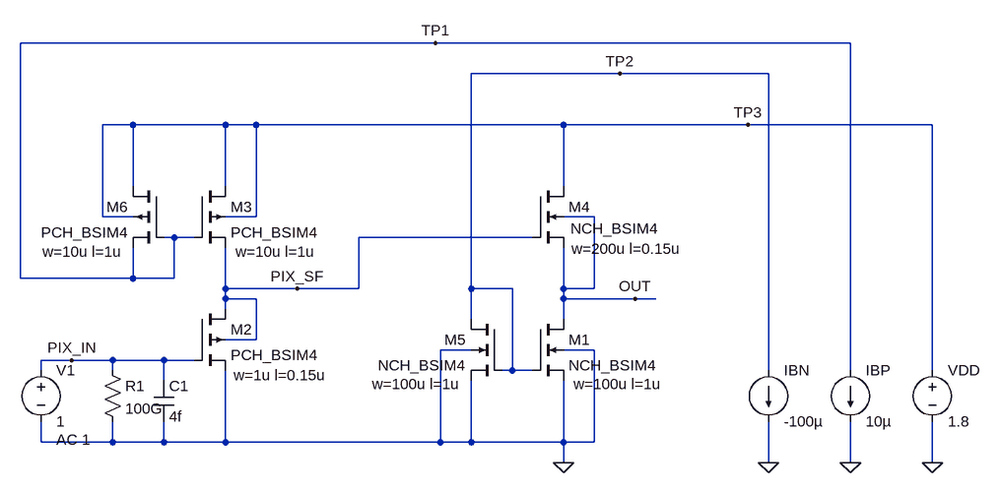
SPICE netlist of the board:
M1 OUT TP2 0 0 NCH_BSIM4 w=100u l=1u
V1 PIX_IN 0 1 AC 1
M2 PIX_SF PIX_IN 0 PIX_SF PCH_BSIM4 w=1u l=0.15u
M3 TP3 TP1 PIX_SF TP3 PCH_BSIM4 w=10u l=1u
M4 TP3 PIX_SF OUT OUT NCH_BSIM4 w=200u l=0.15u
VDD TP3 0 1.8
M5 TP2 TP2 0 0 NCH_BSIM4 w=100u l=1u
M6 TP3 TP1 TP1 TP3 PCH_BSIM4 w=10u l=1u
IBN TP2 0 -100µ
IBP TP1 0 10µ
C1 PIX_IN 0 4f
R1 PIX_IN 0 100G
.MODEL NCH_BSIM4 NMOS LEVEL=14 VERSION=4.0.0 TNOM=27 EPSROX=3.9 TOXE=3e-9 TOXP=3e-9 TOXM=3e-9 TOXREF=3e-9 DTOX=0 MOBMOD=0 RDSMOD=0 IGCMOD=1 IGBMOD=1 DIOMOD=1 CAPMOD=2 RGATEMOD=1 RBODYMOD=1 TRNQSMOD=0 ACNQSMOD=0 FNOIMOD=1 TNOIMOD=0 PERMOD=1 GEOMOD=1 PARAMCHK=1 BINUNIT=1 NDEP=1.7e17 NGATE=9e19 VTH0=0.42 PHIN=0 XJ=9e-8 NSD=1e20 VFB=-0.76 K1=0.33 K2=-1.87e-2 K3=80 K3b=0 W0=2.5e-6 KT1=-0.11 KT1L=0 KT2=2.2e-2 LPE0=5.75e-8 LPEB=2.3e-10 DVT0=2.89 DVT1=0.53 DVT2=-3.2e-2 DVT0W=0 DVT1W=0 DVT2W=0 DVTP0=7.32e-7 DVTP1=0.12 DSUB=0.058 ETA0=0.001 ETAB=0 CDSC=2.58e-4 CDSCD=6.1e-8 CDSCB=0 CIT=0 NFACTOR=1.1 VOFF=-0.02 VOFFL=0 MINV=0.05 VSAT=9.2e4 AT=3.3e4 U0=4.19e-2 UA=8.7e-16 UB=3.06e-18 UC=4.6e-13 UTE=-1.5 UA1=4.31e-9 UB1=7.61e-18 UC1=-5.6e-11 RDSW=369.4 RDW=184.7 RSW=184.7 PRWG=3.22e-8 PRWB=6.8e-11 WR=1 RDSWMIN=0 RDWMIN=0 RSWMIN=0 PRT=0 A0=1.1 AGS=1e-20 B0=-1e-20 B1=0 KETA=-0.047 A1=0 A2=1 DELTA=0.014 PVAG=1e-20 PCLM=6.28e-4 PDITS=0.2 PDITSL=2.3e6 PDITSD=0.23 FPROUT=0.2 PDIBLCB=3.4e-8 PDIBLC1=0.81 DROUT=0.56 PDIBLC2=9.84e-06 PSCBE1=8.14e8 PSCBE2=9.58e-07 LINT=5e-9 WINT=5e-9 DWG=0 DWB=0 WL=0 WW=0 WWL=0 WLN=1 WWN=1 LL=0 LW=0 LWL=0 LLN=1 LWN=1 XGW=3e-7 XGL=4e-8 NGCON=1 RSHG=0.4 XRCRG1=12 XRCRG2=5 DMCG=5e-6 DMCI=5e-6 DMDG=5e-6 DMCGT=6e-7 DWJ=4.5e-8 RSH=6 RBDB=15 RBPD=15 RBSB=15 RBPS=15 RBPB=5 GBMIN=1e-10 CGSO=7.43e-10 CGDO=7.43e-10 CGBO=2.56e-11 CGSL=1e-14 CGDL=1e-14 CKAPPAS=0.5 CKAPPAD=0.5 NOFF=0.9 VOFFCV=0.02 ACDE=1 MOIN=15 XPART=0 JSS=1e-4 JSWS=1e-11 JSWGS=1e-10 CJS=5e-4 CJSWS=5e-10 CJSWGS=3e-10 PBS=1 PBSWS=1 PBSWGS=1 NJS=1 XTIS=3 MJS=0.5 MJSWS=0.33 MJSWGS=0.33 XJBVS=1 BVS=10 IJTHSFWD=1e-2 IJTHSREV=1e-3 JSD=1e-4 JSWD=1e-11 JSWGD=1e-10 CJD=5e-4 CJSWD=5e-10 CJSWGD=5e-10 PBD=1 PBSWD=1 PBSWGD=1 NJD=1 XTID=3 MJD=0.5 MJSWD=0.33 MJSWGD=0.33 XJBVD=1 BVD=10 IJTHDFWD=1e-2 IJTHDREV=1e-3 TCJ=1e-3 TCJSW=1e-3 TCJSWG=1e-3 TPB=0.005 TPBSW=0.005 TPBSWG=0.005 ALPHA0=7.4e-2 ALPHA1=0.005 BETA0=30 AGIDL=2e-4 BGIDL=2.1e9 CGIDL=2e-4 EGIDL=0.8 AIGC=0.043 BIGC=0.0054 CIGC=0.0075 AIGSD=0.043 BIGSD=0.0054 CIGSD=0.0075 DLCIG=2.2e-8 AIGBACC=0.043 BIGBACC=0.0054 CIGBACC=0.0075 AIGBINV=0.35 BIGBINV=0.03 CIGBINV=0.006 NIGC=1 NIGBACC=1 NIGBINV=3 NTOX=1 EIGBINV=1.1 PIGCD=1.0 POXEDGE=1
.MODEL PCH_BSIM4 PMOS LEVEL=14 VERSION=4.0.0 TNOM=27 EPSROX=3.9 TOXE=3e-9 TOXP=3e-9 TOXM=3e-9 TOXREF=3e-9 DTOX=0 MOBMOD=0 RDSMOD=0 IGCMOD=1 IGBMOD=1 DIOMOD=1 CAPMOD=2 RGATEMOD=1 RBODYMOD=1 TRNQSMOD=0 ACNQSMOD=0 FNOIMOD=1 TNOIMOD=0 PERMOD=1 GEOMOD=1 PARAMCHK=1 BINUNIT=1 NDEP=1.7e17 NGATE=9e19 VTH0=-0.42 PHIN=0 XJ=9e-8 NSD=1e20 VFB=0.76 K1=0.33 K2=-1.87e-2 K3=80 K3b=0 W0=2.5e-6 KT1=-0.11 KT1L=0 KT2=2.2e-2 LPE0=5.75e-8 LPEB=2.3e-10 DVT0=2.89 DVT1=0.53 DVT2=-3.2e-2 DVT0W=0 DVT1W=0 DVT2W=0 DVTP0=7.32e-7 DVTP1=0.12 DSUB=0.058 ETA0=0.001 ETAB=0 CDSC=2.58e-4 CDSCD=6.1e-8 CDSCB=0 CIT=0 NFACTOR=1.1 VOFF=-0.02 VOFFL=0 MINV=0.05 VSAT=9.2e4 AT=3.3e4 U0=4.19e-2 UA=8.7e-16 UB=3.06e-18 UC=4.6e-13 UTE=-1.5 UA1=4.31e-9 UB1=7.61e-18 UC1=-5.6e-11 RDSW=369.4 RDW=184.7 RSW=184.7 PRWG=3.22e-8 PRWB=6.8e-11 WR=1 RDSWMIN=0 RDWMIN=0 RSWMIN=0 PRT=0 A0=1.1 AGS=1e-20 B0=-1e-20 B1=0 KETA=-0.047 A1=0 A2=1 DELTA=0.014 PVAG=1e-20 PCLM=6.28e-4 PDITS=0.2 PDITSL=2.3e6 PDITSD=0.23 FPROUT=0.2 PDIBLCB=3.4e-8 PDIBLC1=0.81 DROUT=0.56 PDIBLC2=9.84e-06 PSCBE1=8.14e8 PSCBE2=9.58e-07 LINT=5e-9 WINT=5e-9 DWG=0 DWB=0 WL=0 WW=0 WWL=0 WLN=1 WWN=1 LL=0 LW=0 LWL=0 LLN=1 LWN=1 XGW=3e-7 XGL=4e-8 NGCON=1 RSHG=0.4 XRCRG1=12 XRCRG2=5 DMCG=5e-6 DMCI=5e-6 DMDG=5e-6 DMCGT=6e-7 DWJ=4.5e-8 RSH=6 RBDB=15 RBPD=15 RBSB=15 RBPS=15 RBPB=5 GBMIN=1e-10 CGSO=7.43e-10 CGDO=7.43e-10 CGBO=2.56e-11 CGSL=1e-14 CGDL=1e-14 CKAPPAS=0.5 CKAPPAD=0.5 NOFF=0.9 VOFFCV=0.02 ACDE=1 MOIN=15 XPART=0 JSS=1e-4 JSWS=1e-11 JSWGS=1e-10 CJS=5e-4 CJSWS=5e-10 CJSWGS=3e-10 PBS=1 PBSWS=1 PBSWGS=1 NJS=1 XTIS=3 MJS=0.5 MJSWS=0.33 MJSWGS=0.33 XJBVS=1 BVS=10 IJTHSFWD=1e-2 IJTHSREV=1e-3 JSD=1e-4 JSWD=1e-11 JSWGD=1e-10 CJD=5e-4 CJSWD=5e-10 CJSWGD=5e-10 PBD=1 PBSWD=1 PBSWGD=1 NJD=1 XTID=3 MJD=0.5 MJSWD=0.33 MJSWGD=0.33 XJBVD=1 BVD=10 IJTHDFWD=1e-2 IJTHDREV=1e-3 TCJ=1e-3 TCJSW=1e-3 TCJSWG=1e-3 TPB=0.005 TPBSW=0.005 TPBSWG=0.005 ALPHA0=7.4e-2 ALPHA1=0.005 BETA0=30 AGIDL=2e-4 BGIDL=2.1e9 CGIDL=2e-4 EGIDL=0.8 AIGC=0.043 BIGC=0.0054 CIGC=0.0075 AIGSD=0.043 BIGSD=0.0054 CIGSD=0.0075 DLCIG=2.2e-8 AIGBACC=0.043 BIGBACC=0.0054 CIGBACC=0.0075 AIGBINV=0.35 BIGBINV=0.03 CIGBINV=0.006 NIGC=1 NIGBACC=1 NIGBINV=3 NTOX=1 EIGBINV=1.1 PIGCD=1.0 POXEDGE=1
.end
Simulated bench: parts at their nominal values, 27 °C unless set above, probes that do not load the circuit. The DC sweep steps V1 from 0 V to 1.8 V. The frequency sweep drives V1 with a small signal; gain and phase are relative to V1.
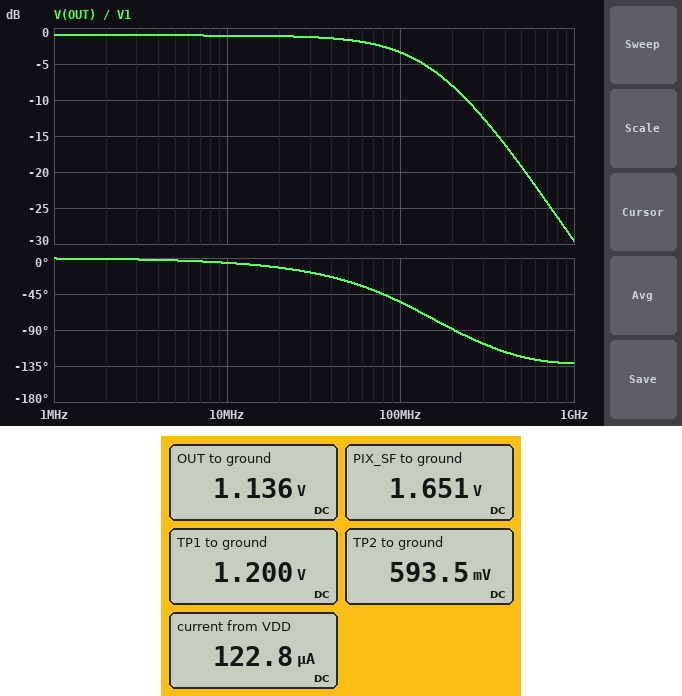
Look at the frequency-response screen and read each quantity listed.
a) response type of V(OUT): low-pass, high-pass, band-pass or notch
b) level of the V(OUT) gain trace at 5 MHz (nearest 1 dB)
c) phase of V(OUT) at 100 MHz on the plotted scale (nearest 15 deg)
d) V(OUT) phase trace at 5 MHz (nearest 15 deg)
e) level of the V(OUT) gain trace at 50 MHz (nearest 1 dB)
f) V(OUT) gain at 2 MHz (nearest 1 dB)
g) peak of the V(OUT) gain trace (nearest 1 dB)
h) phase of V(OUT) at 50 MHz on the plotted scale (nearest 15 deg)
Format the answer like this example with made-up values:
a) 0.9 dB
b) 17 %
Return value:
a) low-pass
b) -1 dB
c) -60 deg
d) 0 deg
e) -2 dB
f) -1 dB
g) -1 dB
h) -30 deg
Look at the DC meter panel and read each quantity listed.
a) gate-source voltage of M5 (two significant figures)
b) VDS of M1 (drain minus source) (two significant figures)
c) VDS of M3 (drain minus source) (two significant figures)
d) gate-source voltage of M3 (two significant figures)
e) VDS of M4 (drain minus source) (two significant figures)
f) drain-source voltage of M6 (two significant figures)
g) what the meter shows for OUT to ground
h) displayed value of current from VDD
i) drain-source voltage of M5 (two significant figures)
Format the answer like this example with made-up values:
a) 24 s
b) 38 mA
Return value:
a) 590 mV
b) 1.1 V
c) 150 mV
d) -450 mV
e) 660 mV
f) 600 mV
g) 1.136 V
h) 122.8 µA
i) 590 mV
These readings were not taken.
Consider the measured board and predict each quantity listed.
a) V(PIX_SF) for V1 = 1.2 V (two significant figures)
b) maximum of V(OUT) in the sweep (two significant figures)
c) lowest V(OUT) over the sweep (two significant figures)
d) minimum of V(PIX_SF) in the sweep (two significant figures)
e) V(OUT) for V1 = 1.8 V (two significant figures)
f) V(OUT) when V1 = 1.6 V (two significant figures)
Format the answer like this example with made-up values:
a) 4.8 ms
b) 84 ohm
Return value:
a) 1.8 V
b) 1.3 V
c) 220 mV
d) 690 mV
e) 1.3 V
f) 1.3 V
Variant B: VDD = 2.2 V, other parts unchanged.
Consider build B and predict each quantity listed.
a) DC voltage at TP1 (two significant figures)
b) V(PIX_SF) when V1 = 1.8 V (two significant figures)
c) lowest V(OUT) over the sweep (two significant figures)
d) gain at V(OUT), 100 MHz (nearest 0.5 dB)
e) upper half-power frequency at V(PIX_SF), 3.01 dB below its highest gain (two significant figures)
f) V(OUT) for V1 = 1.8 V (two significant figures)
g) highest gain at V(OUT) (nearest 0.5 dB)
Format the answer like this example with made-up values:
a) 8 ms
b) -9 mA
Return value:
a) 1.6 V
b) 2.2 V
c) 230 mV
d) -3.0 dB
e) 130 MHz
f) 1.7 V
g) -0.5 dB
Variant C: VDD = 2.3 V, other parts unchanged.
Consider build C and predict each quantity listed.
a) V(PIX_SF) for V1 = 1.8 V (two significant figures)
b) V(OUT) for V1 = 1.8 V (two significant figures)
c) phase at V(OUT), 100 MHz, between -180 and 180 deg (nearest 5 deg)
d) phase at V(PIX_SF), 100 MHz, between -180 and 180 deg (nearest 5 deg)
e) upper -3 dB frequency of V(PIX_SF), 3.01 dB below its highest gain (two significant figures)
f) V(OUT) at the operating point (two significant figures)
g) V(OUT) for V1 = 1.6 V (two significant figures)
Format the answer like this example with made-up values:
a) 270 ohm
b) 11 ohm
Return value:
a) 2.3 V
b) 1.8 V
c) -50 deg
d) -40 deg
e) 130 MHz
f) 1.2 V
g) 1.7 V
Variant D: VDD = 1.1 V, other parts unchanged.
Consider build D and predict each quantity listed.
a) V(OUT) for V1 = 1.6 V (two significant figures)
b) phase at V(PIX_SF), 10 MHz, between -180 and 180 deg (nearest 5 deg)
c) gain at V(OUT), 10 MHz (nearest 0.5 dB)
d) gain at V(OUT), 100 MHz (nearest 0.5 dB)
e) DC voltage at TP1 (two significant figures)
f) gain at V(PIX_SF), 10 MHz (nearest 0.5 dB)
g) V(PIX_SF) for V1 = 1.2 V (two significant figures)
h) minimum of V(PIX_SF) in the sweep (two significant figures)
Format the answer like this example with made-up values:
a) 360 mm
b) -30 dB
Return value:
a) 580 mV
b) 85 deg
c) -68.5 dB
d) -52.0 dB
e) 500 mV
f) -68.0 dB
g) 1.1 V
h) 690 mV
